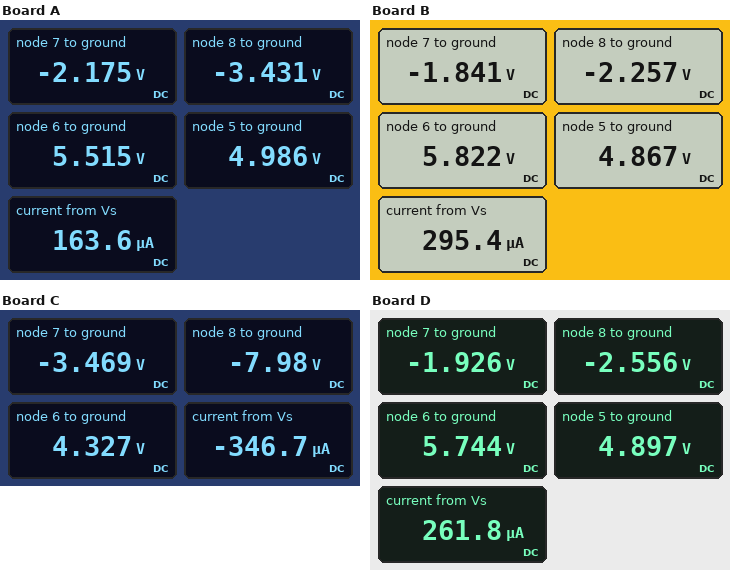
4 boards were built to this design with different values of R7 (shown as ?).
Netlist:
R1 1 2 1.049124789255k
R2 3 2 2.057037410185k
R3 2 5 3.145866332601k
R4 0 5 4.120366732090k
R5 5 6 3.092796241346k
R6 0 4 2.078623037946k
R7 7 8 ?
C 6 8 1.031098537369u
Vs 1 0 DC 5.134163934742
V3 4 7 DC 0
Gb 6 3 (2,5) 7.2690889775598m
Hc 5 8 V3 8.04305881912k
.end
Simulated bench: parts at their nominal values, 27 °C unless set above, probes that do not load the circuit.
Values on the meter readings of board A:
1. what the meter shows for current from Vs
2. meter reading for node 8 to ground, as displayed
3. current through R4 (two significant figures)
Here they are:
163.6 µA
-3.431 V
1.2 mA
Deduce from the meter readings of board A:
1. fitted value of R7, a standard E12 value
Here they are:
1.2 kΩ
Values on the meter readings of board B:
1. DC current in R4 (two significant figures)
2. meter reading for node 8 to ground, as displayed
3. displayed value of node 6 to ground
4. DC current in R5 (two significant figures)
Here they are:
1.2 mA
-2.257 V
5.822 V
310 µA
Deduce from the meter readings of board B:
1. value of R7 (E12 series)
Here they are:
470 Ω
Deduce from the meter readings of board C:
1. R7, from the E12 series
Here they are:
2.7 kΩ
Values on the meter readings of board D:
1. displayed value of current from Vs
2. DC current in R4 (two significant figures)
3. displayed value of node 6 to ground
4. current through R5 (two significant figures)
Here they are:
261.8 µA
1.2 mA
5.744 V
270 µA
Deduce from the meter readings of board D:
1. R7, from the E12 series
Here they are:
680 Ω
